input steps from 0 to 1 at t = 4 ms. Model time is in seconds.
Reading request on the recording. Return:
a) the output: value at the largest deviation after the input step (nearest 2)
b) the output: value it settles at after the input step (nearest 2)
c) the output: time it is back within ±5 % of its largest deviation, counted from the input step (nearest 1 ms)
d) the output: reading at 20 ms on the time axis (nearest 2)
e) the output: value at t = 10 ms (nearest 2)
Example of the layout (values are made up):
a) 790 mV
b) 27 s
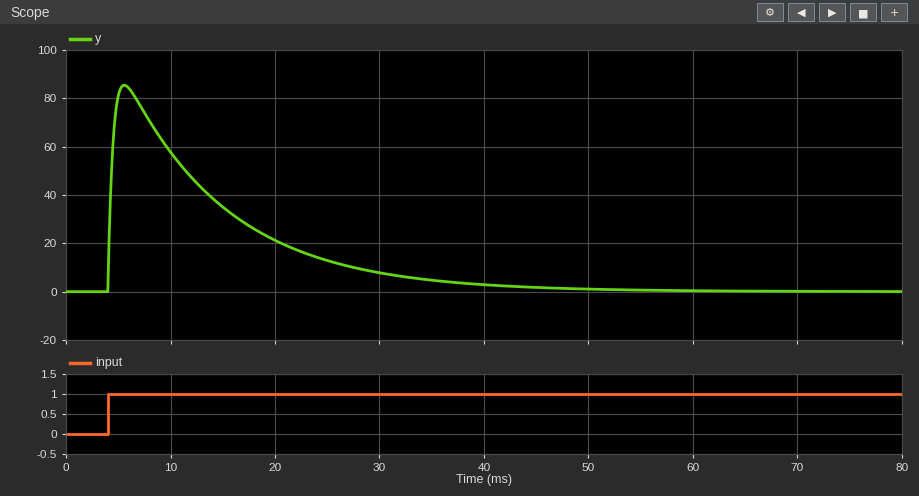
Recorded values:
a) 86
b) 0
c) 32 ms
d) 22
e) 58
